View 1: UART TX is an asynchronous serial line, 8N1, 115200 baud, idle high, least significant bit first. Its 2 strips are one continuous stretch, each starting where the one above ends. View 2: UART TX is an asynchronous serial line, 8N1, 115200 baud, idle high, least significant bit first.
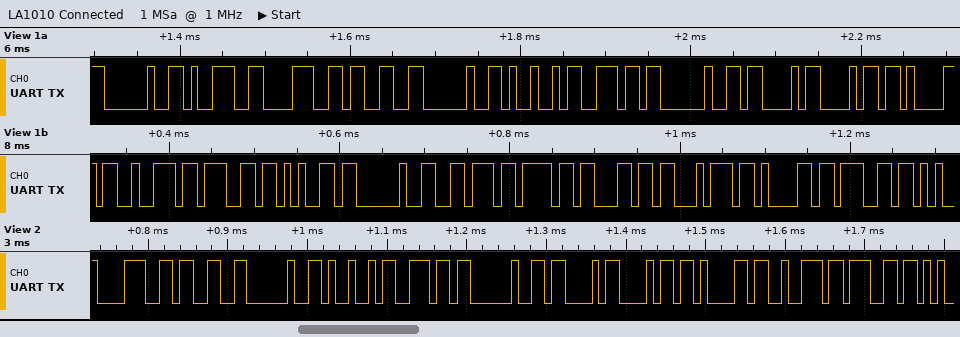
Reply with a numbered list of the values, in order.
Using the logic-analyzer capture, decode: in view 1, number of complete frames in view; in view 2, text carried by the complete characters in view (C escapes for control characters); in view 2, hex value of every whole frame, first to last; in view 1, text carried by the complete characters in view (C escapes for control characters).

1. 21
2. "83 In Charg"
3. 0x38 0x33 0x20 0x49 0x6E 0x20 0x43 0x68 0x61 0x72 0x67
4. " 983 In Charge voltag"
